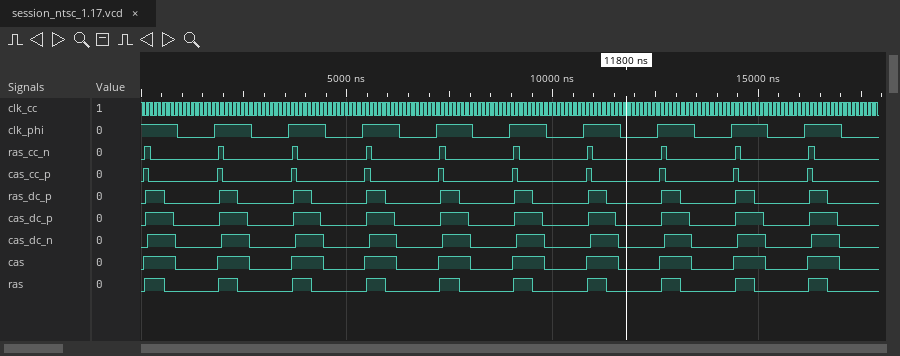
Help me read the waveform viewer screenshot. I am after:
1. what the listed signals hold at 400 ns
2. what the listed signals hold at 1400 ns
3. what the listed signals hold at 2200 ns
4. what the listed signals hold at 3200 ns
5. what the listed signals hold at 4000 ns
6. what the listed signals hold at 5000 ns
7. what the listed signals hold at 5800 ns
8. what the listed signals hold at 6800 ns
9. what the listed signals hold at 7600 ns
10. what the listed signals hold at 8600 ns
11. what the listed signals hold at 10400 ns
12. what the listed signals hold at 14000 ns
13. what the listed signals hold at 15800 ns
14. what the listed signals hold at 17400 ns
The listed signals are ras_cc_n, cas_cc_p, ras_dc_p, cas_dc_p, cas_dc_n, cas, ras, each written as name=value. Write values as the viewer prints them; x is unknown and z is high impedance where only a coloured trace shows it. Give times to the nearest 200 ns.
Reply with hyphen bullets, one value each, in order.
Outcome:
- ras_cc_n=0, cas_cc_p=0, ras_dc_p=1, cas_dc_p=1, cas_dc_n=1, cas=1, ras=1
- ras_cc_n=0, cas_cc_p=0, ras_dc_p=0, cas_dc_p=0, cas_dc_n=0, cas=0, ras=0
- ras_cc_n=0, cas_cc_p=0, ras_dc_p=1, cas_dc_p=1, cas_dc_n=1, cas=1, ras=1
- ras_cc_n=0, cas_cc_p=0, ras_dc_p=0, cas_dc_p=0, cas_dc_n=0, cas=0, ras=0
- ras_cc_n=0, cas_cc_p=0, ras_dc_p=1, cas_dc_p=1, cas_dc_n=1, cas=1, ras=1
- ras_cc_n=0, cas_cc_p=0, ras_dc_p=0, cas_dc_p=0, cas_dc_n=0, cas=0, ras=0
- ras_cc_n=0, cas_cc_p=0, ras_dc_p=1, cas_dc_p=1, cas_dc_n=1, cas=1, ras=1
- ras_cc_n=0, cas_cc_p=0, ras_dc_p=0, cas_dc_p=0, cas_dc_n=0, cas=0, ras=0
- ras_cc_n=0, cas_cc_p=0, ras_dc_p=1, cas_dc_p=1, cas_dc_n=1, cas=1, ras=1
- ras_cc_n=0, cas_cc_p=0, ras_dc_p=0, cas_dc_p=0, cas_dc_n=0, cas=0, ras=0
- ras_cc_n=0, cas_cc_p=0, ras_dc_p=0, cas_dc_p=0, cas_dc_n=0, cas=0, ras=0
- ras_cc_n=0, cas_cc_p=0, ras_dc_p=0, cas_dc_p=0, cas_dc_n=0, cas=0, ras=0
- ras_cc_n=0, cas_cc_p=0, ras_dc_p=0, cas_dc_p=0, cas_dc_n=0, cas=0, ras=0
- ras_cc_n=0, cas_cc_p=0, ras_dc_p=0, cas_dc_p=0, cas_dc_n=0, cas=0, ras=0
